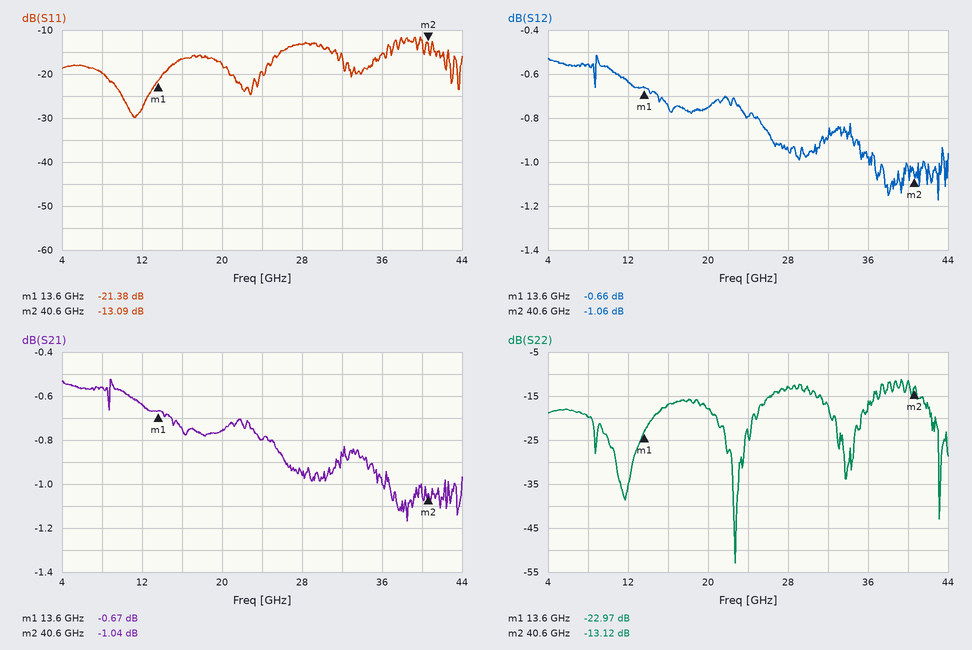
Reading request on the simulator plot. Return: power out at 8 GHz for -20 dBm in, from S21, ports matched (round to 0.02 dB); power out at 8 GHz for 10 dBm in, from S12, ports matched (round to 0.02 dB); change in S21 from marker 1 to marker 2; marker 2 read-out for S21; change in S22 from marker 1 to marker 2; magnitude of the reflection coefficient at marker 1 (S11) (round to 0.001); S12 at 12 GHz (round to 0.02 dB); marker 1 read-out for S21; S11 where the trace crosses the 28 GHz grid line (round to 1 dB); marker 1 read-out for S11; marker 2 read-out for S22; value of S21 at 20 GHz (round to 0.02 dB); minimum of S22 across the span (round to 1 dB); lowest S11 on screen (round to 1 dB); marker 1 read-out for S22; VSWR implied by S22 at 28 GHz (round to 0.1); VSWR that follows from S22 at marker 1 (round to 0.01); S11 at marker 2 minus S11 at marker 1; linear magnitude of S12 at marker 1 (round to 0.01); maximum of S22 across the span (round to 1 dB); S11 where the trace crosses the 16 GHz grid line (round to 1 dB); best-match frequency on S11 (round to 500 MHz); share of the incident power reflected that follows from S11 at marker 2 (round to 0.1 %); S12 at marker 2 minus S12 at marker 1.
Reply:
-20.56 dBm
9.44 dBm
-0.37 dB
-1.04 dB
9.85 dB
0.085
-0.64 dB
-0.67 dB
-13 dB
-21.38 dB
-13.12 dB
-0.76 dB
-53 dB
-30 dB
-22.97 dB
1.6
1.15
8.29 dB
0.93
-11 dB
-17 dB
11.0 GHz
4.9 %
-0.40 dB
